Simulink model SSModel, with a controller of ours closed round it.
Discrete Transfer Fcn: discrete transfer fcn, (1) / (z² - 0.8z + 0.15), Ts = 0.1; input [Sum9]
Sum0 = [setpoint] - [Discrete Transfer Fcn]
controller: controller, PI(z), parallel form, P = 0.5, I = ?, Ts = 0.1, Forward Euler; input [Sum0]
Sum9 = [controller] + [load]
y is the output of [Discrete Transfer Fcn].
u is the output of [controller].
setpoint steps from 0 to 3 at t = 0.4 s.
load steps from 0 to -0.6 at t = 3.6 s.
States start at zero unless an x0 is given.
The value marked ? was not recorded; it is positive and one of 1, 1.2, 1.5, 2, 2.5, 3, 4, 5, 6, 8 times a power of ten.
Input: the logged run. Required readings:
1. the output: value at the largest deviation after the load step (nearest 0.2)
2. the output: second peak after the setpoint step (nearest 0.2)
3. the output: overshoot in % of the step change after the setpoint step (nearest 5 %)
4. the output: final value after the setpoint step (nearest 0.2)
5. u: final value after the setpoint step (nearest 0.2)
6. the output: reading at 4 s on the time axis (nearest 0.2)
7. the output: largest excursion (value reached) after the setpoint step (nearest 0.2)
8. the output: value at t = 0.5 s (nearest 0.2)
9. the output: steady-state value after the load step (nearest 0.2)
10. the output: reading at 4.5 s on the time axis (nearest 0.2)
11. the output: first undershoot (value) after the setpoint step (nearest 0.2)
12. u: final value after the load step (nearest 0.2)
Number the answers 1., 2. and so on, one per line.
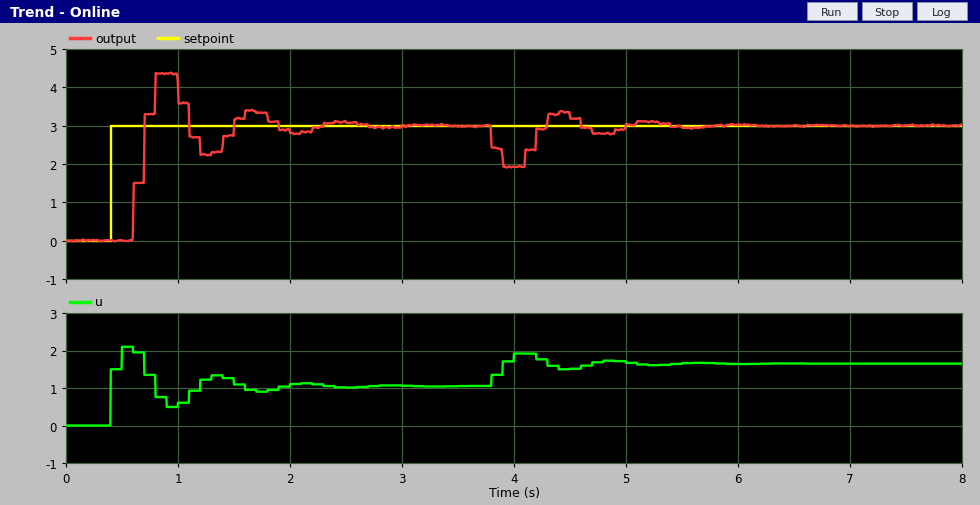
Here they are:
1. 2.0
2. 3.4
3. 45 %
4. 3.0
5. 1.0
6. 2.0
7. 4.4
8. 0.0
9. 3.0
10. 3.2
11. 2.2
12. 1.6
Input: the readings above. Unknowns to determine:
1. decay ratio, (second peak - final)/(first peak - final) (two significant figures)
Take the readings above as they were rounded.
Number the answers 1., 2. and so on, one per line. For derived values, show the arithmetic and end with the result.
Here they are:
1. (3.4 - 3) / (4.4 - 3) = 0.29
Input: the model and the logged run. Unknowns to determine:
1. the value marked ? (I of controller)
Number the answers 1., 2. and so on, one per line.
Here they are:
1. 2
